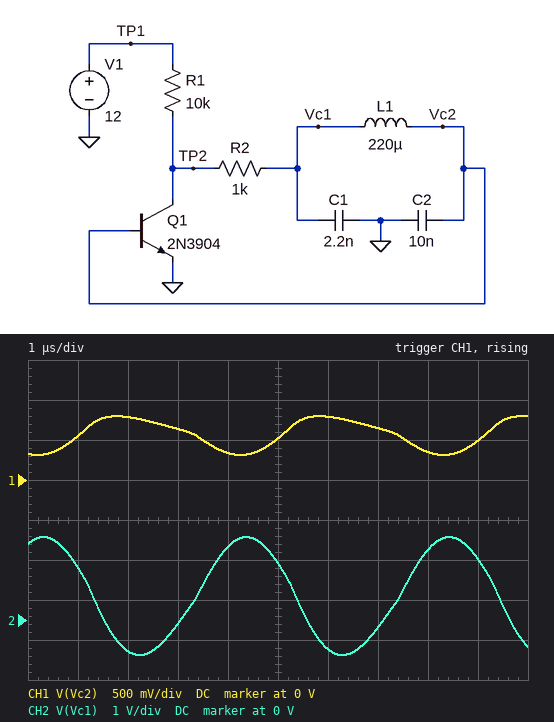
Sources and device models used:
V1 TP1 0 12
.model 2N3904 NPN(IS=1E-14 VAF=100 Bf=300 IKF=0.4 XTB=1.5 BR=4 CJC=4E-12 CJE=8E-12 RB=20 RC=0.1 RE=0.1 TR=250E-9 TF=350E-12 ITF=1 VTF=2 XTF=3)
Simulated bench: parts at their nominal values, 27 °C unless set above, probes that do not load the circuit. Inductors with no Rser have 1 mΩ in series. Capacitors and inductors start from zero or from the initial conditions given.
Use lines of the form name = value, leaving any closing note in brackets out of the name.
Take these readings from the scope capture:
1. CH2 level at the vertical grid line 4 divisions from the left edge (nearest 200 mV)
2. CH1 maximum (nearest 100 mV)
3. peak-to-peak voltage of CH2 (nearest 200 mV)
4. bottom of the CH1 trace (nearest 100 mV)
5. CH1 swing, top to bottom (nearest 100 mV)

CH2 level at the vertical grid line 4 divisions from the left edge = 1.8 V
CH1 maximum = 800 mV
peak-to-peak voltage of CH2 = 3.0 V
bottom of the CH1 trace = 300 mV
CH1 swing, top to bottom = 500 mV
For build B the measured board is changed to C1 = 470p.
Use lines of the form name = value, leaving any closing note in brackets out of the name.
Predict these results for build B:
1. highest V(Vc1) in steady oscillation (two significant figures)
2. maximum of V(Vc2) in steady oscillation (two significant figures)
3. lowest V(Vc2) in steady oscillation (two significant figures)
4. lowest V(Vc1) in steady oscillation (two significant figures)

highest V(Vc1) in steady oscillation = 2.2 V
maximum of V(Vc2) in steady oscillation = 720 mV
lowest V(Vc2) in steady oscillation = 610 mV
lowest V(Vc1) in steady oscillation = -740 mV
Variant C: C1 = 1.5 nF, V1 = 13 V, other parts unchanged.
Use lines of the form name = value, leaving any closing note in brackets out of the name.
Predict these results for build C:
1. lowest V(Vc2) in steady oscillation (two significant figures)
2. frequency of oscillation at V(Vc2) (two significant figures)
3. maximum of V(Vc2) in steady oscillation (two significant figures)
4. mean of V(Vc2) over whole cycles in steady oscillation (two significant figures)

lowest V(Vc2) in steady oscillation = 420 mV
frequency of oscillation at V(Vc2) = 290 kHz
maximum of V(Vc2) in steady oscillation = 790 mV
mean of V(Vc2) over whole cycles in steady oscillation = 620 mV
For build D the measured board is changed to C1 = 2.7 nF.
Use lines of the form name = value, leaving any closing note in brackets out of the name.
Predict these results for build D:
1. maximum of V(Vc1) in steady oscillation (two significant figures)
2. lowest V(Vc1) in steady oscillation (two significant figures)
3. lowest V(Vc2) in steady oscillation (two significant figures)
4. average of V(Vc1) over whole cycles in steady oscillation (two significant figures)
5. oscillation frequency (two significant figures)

maximum of V(Vc1) in steady oscillation = 1.9 V
lowest V(Vc1) in steady oscillation = -790 mV
lowest V(Vc2) in steady oscillation = 250 mV
average of V(Vc1) over whole cycles in steady oscillation = 550 mV
oscillation frequency = 230 kHz
